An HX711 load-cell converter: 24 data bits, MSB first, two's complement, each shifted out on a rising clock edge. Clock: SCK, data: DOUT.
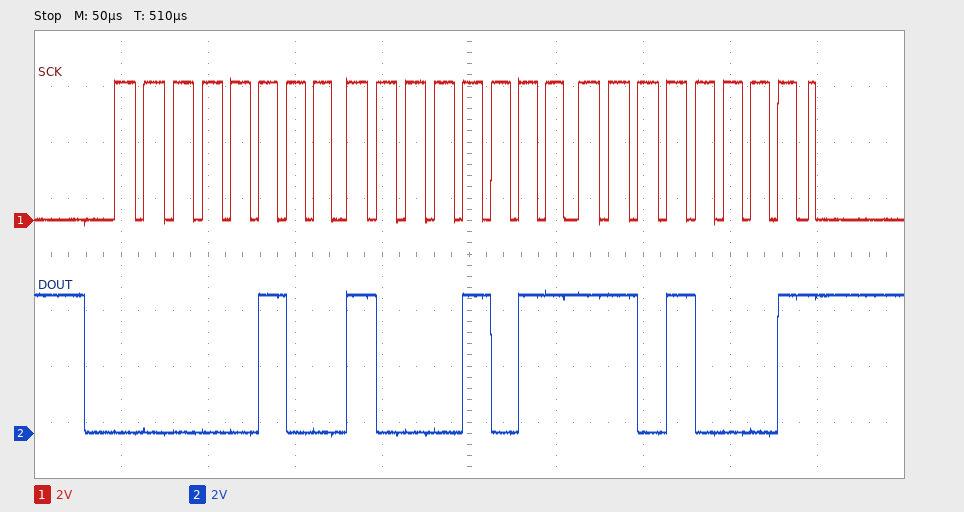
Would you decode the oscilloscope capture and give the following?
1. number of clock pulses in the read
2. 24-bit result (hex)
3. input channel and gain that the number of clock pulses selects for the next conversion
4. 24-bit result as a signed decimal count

25
0x048BD1
channel A, gain 128
297937
